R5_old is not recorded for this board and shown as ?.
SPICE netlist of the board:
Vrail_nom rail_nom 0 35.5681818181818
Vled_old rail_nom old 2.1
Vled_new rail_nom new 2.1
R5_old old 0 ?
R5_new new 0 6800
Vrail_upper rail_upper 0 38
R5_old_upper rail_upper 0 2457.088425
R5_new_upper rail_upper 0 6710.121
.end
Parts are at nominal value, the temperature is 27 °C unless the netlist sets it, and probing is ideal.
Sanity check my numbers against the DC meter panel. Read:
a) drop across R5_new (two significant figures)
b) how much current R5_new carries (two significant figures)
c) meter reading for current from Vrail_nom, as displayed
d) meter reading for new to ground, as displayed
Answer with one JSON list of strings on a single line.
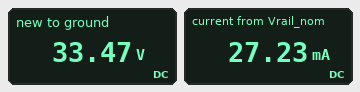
["33 V", "4.9 mA", "27.23 mA", "33.47 V"]
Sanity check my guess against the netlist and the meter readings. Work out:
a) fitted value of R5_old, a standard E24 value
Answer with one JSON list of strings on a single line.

["1.5 kΩ"]
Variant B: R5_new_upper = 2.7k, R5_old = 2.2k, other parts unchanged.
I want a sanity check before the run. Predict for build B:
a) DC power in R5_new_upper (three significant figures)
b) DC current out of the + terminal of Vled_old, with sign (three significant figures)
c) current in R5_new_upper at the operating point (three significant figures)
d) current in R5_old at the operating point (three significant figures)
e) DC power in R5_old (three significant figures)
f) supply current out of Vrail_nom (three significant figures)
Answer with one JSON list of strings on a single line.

["535 mW", "-15.2 mA", "14.1 mA", "15.2 mA", "509 mW", "20.1 mA"]
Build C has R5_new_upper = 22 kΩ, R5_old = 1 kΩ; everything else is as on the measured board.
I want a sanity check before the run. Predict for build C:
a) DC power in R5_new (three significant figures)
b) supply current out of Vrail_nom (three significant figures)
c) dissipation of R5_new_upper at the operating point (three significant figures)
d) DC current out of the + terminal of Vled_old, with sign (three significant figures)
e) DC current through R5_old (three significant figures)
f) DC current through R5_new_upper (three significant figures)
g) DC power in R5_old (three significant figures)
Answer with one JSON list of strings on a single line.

["165 mW", "38.4 mA", "65.6 mW", "-33.5 mA", "33.5 mA", "1.73 mA", "1.12 W"]
